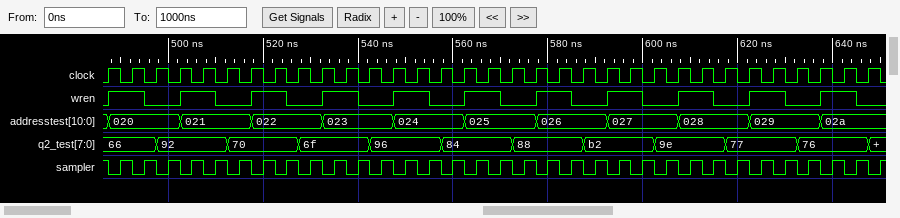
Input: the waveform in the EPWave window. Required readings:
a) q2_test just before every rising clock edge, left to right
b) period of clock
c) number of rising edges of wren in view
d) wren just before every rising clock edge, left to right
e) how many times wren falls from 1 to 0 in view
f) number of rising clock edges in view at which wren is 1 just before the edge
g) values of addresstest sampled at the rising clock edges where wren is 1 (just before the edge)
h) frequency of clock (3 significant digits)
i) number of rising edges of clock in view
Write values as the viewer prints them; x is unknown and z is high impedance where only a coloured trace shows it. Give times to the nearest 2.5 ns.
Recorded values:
66, 66, 66, 92, 92, 92, 70, 70, 70, 6f, 6f, 6f, 96, 96, 96, 84, 84, 84, 88, 88, 88, b2, b2, b2, 9e, 9e, 9e, 77, 77, 77, 76, 76, 76
5 ns
11
0 1 0 0 1 0 0 1 0 0 1 0 0 1 0 0 1 0 0 1 0 0 1 0 0 1 0 0 1 0 0 1 0
11
11
020, 021, 022, 023, 024, 025, 026, 027, 028, 029, 02a
200 MHz
33
